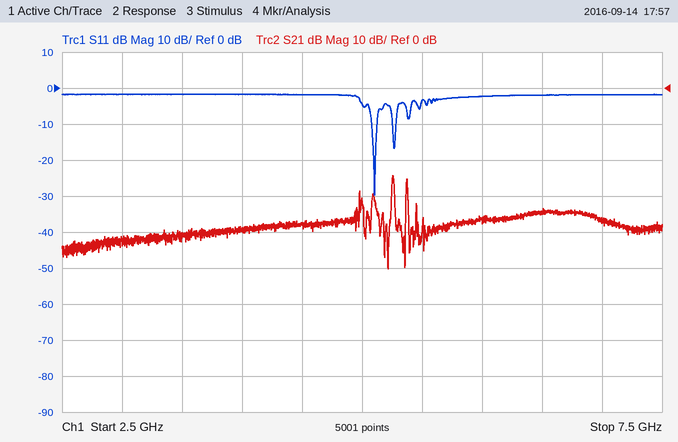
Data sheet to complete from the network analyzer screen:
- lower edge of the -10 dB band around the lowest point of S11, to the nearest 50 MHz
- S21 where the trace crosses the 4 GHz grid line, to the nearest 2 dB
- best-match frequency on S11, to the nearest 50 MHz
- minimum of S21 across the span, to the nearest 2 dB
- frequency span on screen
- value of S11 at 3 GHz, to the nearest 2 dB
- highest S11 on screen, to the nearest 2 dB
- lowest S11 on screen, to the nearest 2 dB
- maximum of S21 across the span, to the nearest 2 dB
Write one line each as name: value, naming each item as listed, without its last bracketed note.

lower edge of the -10 dB band around the lowest point of S11, to the nearest 50 MHz: 5.10 GHz
S21 where the trace crosses the 4 GHz grid line, to the nearest 2 dB: -40 dB
best-match frequency on S11, to the nearest 50 MHz: 5.10 GHz
minimum of S21 across the span, to the nearest 2 dB: -50 dB
frequency span on screen: 5 GHz
value of S11 at 3 GHz, to the nearest 2 dB: -2 dB
highest S11 on screen, to the nearest 2 dB: -2 dB
lowest S11 on screen, to the nearest 2 dB: -30 dB
maximum of S21 across the span, to the nearest 2 dB: -24 dB
